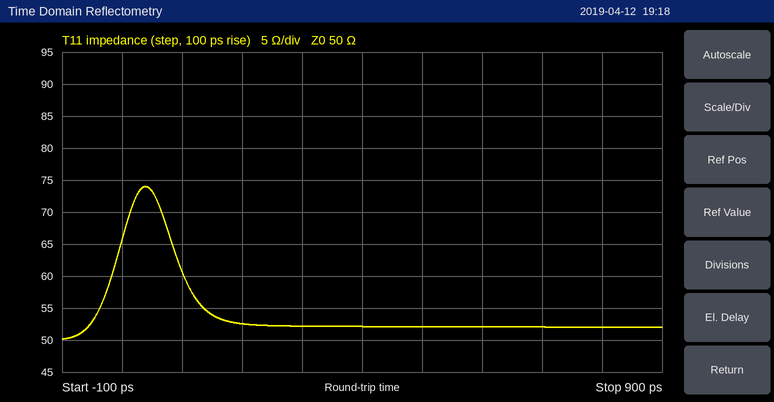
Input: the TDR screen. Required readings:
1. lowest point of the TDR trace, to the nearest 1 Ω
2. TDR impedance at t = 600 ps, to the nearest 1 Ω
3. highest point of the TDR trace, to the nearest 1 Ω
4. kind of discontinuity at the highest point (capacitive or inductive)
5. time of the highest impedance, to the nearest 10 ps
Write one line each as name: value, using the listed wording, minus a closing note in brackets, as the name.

lowest point of the TDR trace, to the nearest 1 Ω: 50 Ω
TDR impedance at t = 600 ps, to the nearest 1 Ω: 52 Ω
highest point of the TDR trace, to the nearest 1 Ω: 74 Ω
kind of discontinuity at the highest point: inductive
time of the highest impedance, to the nearest 10 ps: 40 ps
